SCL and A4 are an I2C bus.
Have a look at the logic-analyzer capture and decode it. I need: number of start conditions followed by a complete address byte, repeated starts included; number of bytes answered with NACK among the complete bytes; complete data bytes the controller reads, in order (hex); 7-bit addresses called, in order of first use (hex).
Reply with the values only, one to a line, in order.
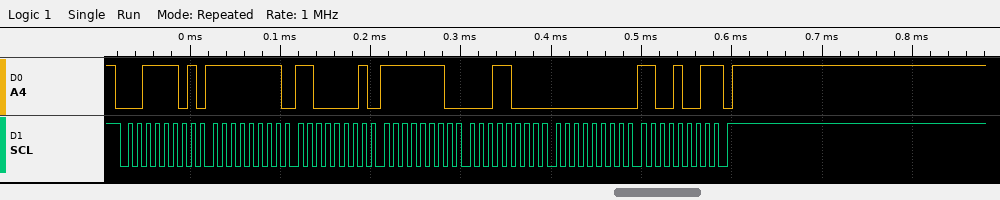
1
1
FF C1 FE 18 00 C9
0x1E
